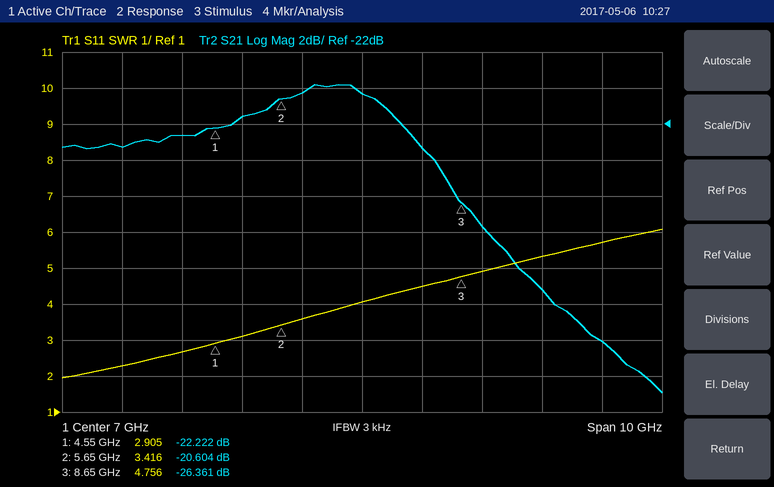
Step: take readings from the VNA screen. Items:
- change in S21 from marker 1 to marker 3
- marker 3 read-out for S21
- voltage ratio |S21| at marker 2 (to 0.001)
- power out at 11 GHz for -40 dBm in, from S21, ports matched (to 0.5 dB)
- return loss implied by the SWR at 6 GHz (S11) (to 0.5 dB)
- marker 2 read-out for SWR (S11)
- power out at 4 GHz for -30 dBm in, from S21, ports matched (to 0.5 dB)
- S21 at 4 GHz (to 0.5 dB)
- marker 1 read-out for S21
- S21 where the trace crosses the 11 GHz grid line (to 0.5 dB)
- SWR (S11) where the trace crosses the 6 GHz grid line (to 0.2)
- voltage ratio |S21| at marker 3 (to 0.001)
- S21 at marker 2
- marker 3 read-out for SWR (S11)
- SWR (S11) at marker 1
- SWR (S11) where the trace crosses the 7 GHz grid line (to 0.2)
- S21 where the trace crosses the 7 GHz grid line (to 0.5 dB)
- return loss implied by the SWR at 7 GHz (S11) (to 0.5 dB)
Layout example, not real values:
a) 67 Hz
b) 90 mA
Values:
a) -4.139 dB
b) -26.361 dB
c) 0.093
d) -74.0 dBm
e) 5.0 dB
f) 3.416
g) -52.5 dBm
h) -22.5 dB
i) -22.222 dB
j) -34.0 dB
k) 3.6
l) 0.048
m) -20.604 dB
n) 4.756
o) 2.905
p) 4.0
q) -20.5 dB
r) 4.5 dB
